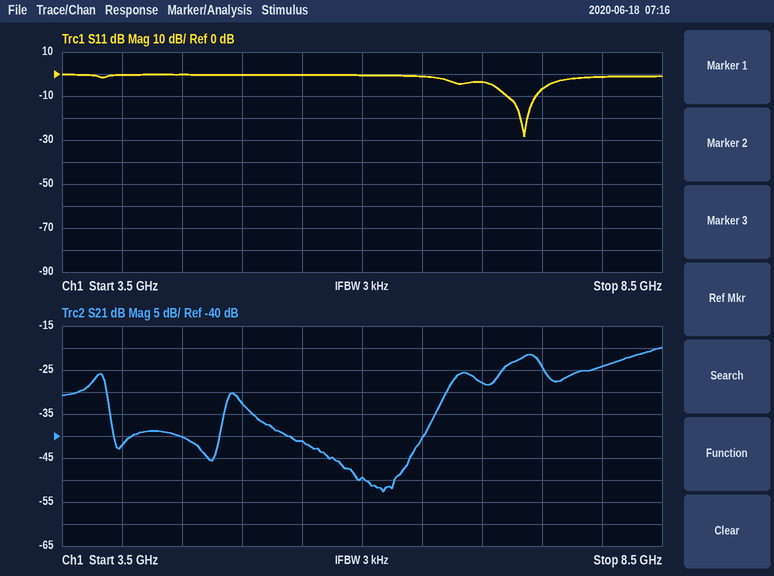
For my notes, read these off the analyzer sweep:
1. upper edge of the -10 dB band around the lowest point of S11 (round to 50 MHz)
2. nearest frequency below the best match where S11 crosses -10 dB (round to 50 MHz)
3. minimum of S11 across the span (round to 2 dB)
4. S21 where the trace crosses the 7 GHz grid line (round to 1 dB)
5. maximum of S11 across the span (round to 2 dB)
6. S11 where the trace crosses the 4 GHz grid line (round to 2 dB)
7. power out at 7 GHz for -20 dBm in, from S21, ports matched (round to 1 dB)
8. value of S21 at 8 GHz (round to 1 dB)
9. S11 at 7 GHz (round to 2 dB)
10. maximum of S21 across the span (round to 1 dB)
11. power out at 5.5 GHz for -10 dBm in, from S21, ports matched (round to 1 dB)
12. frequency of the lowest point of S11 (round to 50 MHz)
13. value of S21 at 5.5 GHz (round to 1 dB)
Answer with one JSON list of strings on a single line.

["7.45 GHz", "7.20 GHz", "-28 dB", "-28 dB", "0 dB", "0 dB", "-48 dBm", "-24 dB", "-4 dB", "-20 dB", "-51 dBm", "7.35 GHz", "-41 dB"]
